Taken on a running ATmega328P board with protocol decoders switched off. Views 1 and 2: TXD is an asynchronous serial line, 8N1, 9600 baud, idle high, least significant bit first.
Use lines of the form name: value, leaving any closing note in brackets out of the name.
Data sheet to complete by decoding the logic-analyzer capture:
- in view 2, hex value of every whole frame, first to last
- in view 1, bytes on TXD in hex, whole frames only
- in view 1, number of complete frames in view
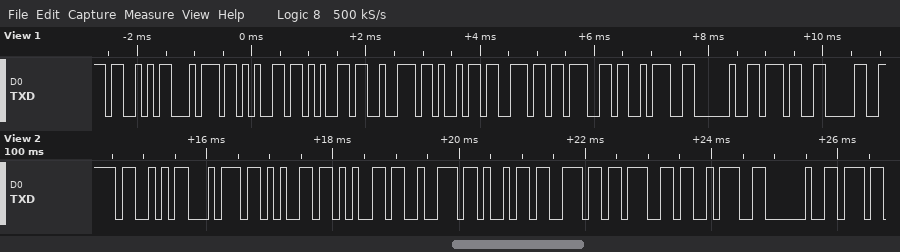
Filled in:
in view 2, hex value of every whole frame, first to last: 0x53 0x74 0x65 0x65 0x72 0x69 0x6E 0x67 0x3A 0x20
in view 1, bytes on TXD in hex, whole frames only: 53 74 65 65 72 69 6E 67 3A 20 37 30
in view 1, number of complete frames in view: 12
